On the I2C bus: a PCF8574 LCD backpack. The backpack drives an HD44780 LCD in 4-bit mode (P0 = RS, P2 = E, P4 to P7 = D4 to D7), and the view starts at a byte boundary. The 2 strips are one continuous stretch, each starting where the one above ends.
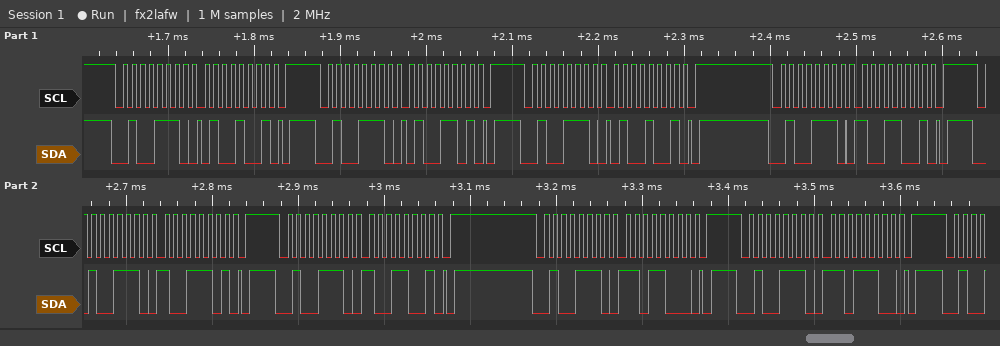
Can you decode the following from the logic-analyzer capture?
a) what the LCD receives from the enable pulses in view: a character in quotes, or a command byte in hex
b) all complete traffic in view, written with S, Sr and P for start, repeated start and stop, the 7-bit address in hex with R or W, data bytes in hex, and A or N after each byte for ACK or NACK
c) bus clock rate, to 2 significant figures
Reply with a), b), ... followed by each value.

a) 'I'
b) S 27W A 49 A P S 27W A 4D A P S 27W A 49 A P S 27W A 99 A P S 27W A 9D A P S 27W A 99 A P S 27W A D8 A P S 27W A DC A P
c) 100 kHz
